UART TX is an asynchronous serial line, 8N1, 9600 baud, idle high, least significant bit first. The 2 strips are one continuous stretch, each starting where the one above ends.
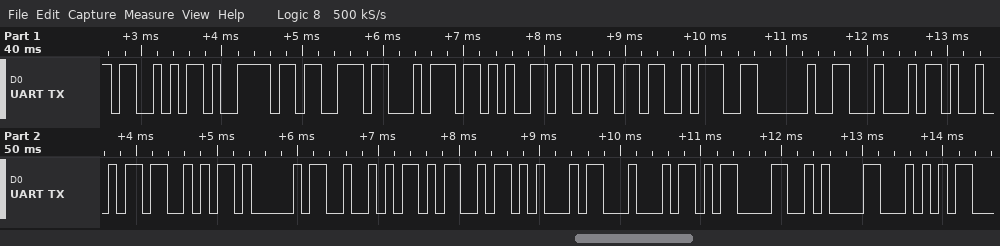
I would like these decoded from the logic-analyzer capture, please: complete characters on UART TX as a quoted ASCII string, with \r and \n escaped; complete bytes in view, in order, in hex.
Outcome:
"System: DISARMED\r\nT"
53 79 73 74 65 6D 3A 20 44 49 53 41 52 4D 45 44 0D 0A 54
